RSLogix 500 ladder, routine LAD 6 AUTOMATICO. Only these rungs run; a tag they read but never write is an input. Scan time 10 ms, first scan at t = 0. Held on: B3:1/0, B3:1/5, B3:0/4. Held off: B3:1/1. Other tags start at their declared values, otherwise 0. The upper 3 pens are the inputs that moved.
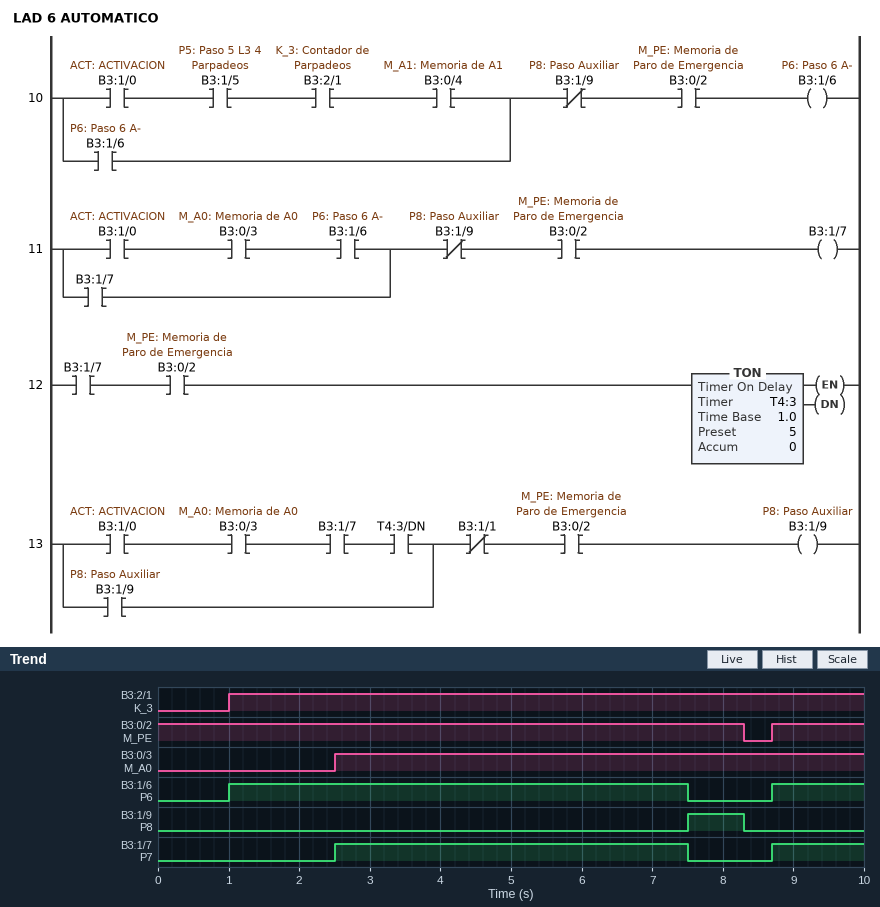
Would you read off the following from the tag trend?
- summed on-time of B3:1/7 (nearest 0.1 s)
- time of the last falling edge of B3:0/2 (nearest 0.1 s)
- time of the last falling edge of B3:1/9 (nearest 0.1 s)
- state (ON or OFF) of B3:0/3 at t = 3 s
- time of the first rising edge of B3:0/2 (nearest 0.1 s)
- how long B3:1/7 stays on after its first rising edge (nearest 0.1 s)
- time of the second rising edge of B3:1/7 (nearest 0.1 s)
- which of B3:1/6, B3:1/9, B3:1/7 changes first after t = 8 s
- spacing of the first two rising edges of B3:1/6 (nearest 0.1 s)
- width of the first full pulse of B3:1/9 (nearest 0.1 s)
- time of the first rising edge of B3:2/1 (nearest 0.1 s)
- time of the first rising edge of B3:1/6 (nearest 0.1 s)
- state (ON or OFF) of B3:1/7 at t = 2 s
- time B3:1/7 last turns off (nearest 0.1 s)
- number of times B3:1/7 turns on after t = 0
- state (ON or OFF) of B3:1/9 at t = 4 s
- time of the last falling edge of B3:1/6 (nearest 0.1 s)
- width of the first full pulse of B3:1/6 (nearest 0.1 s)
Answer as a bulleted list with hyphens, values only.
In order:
- 6.3 s
- 8.3 s
- 8.3 s
- ON
- 8.7 s
- 5.0 s
- 8.7 s
- B3:1/9
- 7.7 s
- 0.8 s
- 1.0 s
- 1.0 s
- OFF
- 7.5 s
- 2
- OFF
- 7.5 s
- 6.5 s
